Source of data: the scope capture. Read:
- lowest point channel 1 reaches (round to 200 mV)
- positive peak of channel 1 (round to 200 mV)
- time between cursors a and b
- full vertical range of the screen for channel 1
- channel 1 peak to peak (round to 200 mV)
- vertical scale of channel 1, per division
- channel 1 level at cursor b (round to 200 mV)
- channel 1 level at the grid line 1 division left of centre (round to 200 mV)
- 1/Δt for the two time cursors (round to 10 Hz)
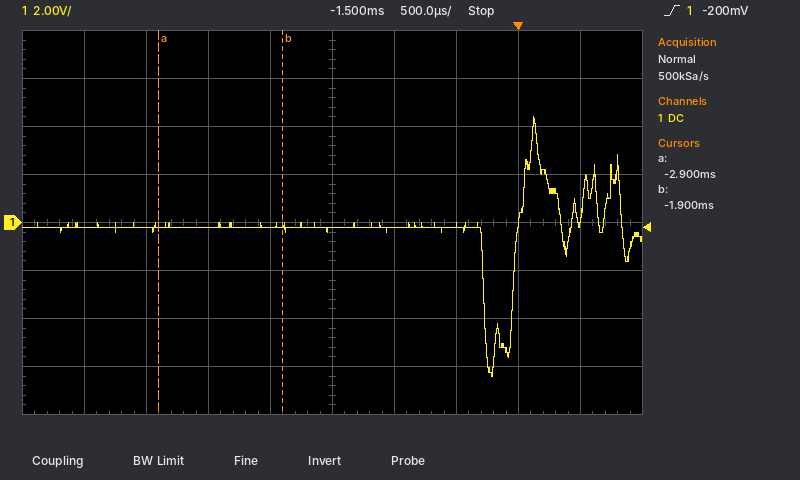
-6.4 V
4.4 V
1.00 ms
16 V
10.8 V
2 V
-200 mV
-200 mV
1.00 kHz
